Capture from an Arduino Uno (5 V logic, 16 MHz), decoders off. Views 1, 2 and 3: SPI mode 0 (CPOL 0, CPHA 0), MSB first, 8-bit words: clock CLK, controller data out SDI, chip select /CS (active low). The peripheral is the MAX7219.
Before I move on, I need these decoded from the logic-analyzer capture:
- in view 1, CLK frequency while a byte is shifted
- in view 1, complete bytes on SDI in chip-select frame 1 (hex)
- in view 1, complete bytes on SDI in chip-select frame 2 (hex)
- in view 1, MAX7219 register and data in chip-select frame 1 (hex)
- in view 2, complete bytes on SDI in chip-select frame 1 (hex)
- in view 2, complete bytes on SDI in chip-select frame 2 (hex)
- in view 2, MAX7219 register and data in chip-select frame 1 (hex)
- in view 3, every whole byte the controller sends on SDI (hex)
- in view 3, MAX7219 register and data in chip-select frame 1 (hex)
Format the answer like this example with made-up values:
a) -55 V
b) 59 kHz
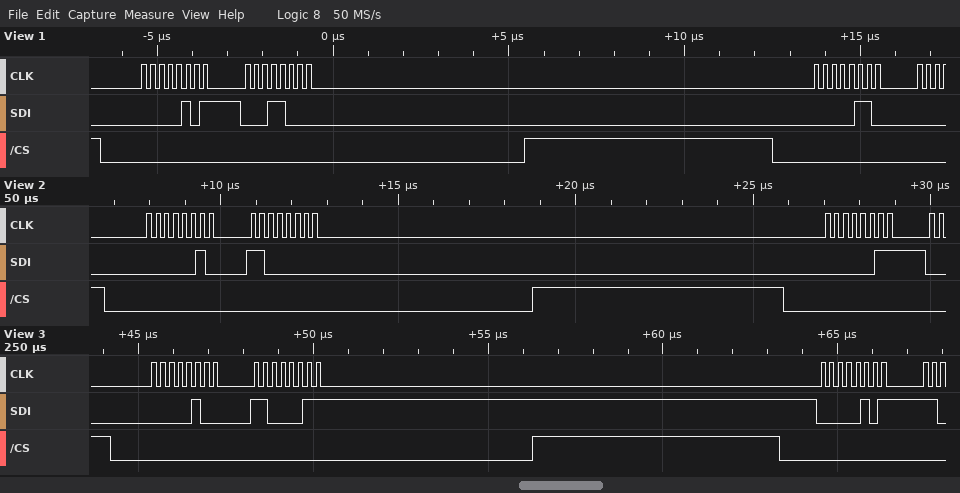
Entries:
a) 4 MHz
b) 0x05 0x18
c) 0x06
d) register 0x5, data 0x18
e) 02 C0
f) 03
g) register 0x2, data 0xC0
h) 04 C3 05
i) register 0x4, data 0xC3
